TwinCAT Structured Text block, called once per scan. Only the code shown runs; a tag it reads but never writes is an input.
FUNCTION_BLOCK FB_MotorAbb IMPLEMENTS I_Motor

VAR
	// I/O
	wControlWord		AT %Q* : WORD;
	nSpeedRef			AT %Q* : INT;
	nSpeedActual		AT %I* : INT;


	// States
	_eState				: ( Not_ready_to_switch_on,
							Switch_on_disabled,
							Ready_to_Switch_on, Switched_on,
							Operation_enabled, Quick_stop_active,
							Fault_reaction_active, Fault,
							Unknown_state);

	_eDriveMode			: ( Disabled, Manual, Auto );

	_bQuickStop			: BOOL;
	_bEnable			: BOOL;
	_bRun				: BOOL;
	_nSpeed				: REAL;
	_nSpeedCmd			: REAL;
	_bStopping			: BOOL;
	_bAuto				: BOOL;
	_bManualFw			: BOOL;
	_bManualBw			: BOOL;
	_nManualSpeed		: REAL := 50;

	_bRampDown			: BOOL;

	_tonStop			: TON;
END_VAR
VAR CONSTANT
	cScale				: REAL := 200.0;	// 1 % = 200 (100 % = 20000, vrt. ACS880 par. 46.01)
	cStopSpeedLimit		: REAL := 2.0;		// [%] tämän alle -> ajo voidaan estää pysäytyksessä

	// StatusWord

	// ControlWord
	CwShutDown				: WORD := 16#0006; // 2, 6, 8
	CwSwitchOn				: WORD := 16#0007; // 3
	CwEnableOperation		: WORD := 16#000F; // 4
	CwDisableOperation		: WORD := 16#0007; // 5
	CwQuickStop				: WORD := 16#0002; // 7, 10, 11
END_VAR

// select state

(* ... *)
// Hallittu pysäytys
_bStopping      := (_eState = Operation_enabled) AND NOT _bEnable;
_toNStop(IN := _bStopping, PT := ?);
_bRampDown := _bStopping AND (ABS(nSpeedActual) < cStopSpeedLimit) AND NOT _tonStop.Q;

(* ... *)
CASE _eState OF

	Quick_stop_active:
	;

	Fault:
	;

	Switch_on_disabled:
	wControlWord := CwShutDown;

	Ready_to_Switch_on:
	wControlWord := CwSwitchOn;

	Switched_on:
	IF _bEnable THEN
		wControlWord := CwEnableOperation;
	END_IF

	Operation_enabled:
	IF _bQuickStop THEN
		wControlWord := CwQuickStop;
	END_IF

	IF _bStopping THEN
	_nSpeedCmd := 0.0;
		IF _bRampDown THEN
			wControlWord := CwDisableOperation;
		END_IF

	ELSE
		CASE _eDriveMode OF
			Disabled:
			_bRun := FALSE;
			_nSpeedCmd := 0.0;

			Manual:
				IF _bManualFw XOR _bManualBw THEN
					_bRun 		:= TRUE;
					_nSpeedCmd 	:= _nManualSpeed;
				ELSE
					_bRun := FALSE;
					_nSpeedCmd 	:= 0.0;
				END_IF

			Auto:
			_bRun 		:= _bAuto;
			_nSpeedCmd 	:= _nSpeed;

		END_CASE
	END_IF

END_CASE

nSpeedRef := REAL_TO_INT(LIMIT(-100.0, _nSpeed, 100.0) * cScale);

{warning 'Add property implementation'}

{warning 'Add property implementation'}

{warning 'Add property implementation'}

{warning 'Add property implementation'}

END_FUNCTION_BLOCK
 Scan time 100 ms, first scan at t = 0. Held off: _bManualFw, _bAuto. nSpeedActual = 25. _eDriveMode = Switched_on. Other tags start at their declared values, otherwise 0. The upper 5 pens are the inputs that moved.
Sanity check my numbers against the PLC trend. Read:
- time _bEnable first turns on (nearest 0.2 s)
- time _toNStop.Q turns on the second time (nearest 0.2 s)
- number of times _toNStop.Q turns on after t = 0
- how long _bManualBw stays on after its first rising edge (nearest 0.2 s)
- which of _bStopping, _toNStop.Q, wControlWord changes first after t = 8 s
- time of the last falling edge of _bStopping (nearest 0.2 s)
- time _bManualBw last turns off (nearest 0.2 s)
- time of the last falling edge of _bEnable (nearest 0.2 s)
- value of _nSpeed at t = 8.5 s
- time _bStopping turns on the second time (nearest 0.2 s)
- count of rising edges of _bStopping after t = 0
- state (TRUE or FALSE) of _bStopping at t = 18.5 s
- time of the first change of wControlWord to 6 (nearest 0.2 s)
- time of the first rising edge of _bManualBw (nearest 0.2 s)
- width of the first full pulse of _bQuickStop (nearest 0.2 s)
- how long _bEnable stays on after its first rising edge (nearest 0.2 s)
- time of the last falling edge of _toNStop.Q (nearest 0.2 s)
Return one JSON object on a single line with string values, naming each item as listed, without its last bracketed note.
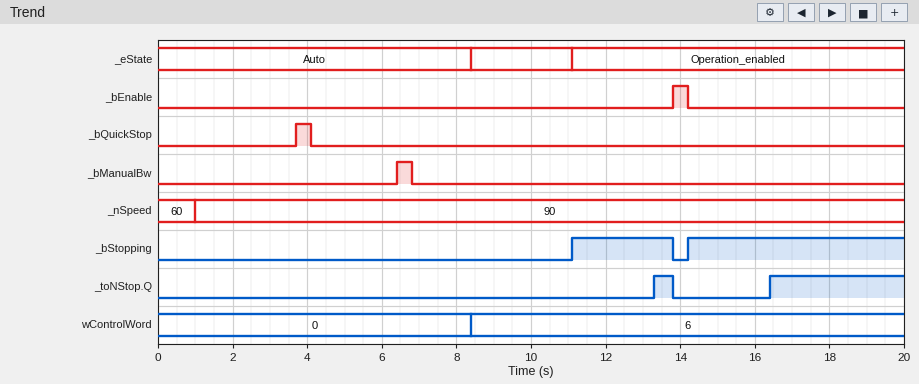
{"time _bEnable first turns on": "13.8 s", "time _toNStop.Q turns on the second time": "16.4 s", "number of times _toNStop.Q turns on after t = 0": "2", "how long _bManualBw stays on after its first rising edge": "0.4 s", "which of _bStopping, _toNStop.Q, wControlWord changes first after t = 8 s": "wControlWord", "time of the last falling edge of _bStopping": "13.8 s", "time _bManualBw last turns off": "6.8 s", "time of the last falling edge of _bEnable": "14.2 s", "value of _nSpeed at t = 8.5 s": "90", "time _bStopping turns on the second time": "14.2 s", "count of rising edges of _bStopping after t = 0": "2", "state (TRUE or FALSE) of _bStopping at t = 18.5 s": "TRUE", "time of the first change of wControlWord to 6": "8.4 s", "time of the first rising edge of _bManualBw": "6.4 s", "width of the first full pulse of _bQuickStop": "0.4 s", "how long _bEnable stays on after its first rising edge": "0.4 s", "time of the last falling edge of _toNStop.Q": "13.8 s"}
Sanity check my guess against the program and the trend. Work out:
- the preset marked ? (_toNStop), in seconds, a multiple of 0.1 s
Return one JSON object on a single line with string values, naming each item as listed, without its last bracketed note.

{"the preset marked ? (_toNStop), in seconds, a multiple of 0.1 s": "2.2 s"}
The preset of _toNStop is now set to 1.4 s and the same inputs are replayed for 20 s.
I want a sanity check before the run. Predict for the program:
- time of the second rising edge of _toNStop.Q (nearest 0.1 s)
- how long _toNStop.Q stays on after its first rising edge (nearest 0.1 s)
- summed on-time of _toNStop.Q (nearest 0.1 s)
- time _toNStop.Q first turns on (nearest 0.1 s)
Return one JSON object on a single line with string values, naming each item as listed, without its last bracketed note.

{"time of the second rising edge of _toNStop.Q": "15.6 s", "how long _toNStop.Q stays on after its first rising edge": "1.3 s", "summed on-time of _toNStop.Q": "5.7 s", "time _toNStop.Q first turns on": "12.5 s"}
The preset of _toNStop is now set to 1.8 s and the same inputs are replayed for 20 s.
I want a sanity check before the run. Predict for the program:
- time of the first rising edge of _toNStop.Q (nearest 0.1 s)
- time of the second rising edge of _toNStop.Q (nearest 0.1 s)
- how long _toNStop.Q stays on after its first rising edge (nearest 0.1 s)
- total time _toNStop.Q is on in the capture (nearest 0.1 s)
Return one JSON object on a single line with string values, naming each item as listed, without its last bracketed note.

{"time of the first rising edge of _toNStop.Q": "12.9 s", "time of the second rising edge of _toNStop.Q": "16.0 s", "how long _toNStop.Q stays on after its first rising edge": "0.9 s", "total time _toNStop.Q is on in the capture": "4.9 s"}
